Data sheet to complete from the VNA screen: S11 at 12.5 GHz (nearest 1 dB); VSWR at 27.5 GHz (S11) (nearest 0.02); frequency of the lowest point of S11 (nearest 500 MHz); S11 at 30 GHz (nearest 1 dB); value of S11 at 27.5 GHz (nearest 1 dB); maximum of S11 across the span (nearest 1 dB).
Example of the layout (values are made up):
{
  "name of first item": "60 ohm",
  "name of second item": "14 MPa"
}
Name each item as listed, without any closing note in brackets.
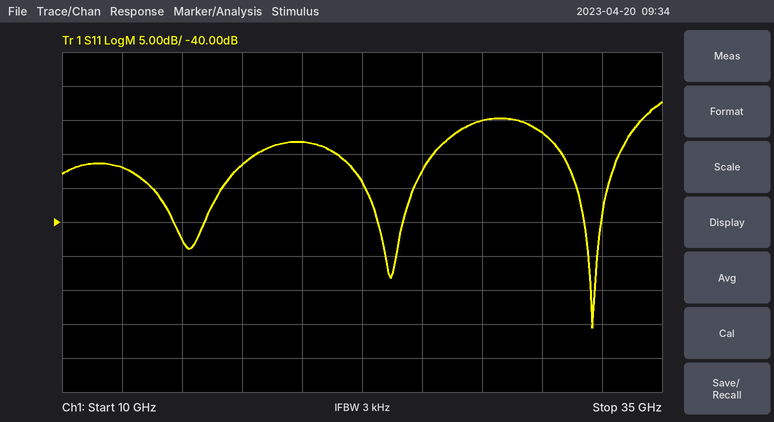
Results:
{
  "S11 at 12.5 GHz": "-32 dB",
  "VSWR at 27.5 GHz (S11)": "1.12",
  "frequency of the lowest point of S11": "32.0 GHz",
  "S11 at 30 GHz": "-27 dB",
  "value of S11 at 27.5 GHz": "-25 dB",
  "maximum of S11 across the span": "-22 dB"
}
